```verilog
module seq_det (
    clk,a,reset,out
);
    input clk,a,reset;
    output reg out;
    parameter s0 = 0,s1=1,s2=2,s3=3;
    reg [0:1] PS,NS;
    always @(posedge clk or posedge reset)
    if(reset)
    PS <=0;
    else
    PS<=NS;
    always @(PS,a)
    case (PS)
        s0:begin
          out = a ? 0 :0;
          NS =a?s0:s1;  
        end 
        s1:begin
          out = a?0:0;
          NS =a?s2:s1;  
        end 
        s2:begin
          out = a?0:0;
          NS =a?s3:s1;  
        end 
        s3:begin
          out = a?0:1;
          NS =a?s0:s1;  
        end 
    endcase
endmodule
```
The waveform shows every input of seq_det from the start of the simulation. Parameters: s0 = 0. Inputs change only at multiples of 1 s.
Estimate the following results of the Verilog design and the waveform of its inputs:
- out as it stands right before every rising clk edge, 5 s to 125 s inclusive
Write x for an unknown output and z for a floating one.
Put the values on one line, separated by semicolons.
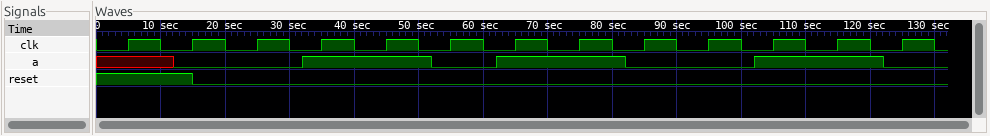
0 0 0 0 0 1 0 0 1 0 0 0 1
